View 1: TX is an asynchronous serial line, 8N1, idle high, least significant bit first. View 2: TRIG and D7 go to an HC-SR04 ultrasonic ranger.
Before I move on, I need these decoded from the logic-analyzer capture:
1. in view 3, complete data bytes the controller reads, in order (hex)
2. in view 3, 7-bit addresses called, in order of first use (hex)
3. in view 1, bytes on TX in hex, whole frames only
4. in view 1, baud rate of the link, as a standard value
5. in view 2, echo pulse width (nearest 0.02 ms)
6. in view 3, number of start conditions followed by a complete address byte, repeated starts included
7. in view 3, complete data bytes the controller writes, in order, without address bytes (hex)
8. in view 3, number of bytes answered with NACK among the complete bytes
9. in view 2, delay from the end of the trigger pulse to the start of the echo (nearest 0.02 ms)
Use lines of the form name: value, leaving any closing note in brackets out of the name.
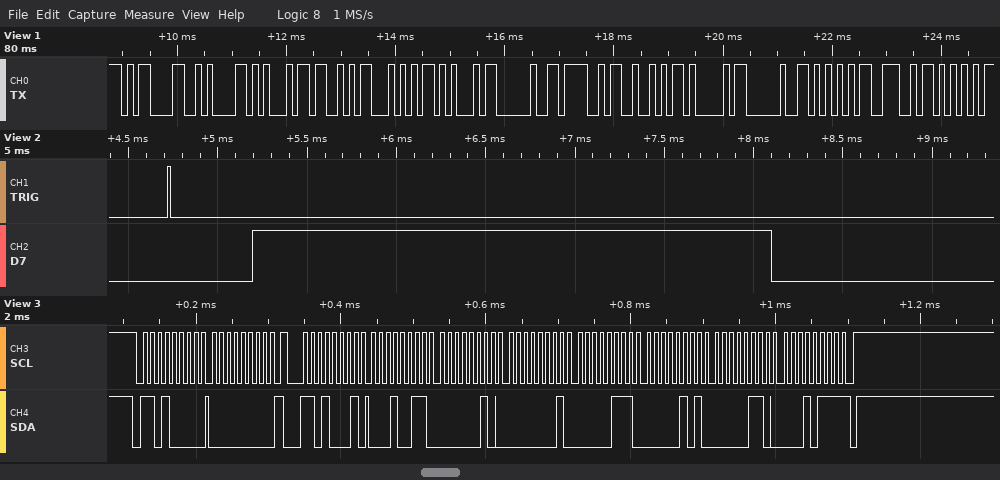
in view 3, complete data bytes the controller reads, in order: 13 02 01 07 05 06 17
in view 3, 7-bit addresses called, in order of first use: 0x68
in view 1, bytes on TX in hex, whole frames only: 0D 0A 45 53 54 45 20 4F 52 41 20 55 4E 55
in view 1, baud rate of the link, as a standard value: 9600 baud
in view 2, echo pulse width: 2.90 ms
in view 3, number of start conditions followed by a complete address byte, repeated starts included: 2
in view 3, complete data bytes the controller writes, in order, without address bytes: 00
in view 3, number of bytes answered with NACK among the complete bytes: 1
in view 2, delay from the end of the trigger pulse to the start of the echo: 0.46 ms
